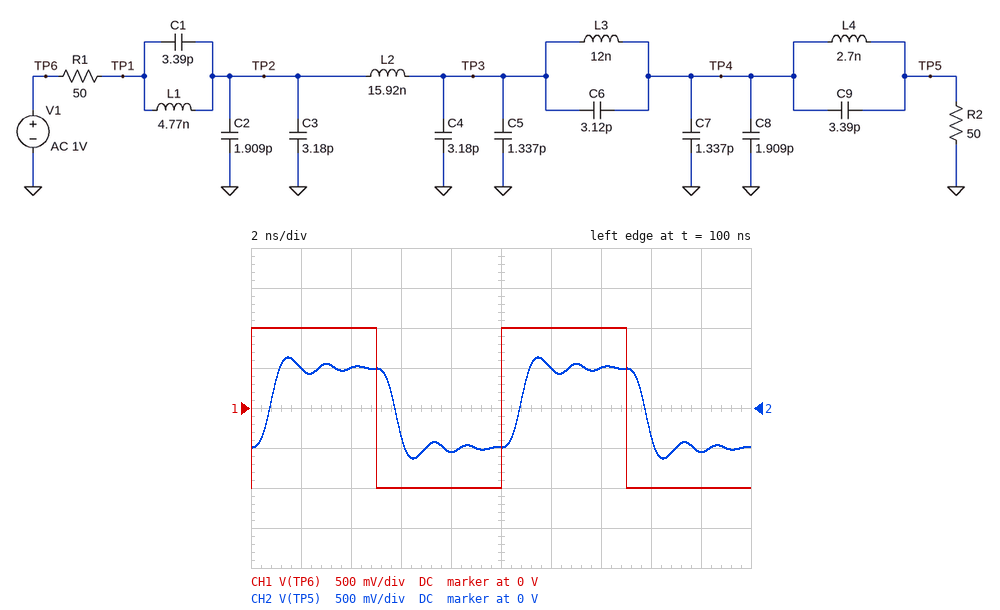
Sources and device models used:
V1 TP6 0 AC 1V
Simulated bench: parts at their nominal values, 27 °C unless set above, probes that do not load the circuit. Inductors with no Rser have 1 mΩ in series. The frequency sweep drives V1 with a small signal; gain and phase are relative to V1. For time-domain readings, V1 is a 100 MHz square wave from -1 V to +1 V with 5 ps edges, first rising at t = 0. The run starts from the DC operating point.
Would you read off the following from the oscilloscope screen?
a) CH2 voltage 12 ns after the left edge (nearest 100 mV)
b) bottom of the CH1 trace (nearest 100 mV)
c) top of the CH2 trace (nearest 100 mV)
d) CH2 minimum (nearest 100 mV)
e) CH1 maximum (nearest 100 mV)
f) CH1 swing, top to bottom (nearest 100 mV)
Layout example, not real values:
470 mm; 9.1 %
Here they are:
500 mV; -1.0 V; 600 mV; -600 mV; 1.0 V; 2.0 V
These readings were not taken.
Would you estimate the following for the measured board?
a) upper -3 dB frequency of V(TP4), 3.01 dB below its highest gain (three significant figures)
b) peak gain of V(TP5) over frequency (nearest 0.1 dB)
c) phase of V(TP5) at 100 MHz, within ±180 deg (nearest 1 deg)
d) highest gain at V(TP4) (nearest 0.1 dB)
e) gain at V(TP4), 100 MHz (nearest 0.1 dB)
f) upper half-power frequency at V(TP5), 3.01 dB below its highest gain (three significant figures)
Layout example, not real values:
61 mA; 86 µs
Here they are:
673 MHz; -6.0 dB; -24 deg; -6.0 dB; -6.0 dB; 666 MHz
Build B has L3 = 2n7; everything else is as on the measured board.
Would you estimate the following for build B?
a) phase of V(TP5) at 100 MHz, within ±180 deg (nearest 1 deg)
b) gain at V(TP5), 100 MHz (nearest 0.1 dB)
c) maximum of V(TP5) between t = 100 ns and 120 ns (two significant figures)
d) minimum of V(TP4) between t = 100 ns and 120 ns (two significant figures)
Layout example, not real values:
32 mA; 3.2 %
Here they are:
-21 deg; -6.0 dB; 660 mV; -660 mV
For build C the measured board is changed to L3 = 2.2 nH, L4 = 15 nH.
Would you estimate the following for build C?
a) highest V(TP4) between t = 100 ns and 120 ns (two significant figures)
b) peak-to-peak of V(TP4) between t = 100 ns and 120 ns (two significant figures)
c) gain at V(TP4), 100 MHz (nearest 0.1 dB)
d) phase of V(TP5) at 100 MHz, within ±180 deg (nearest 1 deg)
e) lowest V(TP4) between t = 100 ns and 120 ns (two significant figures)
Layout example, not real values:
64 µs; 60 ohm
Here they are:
920 mV; 1.8 V; -5.9 dB; -25 deg; -920 mV
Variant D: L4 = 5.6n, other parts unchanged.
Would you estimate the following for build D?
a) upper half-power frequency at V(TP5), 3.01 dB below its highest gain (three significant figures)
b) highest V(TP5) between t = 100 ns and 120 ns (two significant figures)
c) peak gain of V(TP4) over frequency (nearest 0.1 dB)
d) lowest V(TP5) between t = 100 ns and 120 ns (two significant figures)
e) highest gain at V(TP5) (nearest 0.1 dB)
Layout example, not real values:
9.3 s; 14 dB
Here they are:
693 MHz; 650 mV; -5.7 dB; -650 mV; -6.0 dB
